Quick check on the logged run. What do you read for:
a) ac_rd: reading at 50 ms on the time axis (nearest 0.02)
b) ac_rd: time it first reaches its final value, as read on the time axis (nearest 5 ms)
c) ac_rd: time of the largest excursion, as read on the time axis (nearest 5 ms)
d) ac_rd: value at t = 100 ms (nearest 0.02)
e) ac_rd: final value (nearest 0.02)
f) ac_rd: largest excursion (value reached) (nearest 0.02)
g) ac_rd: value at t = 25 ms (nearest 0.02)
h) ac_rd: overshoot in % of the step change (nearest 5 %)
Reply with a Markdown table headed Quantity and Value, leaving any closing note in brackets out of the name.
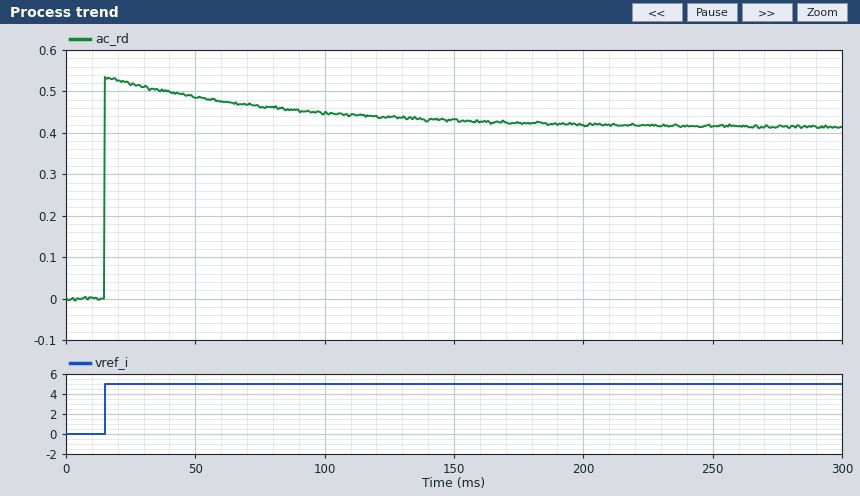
| Quantity | Value |
|---|---|
| ac_rd: reading at 50 ms on the time axis | 0.48 |
| ac_rd: time it first reaches its final value, as read on the time axis | 15 ms |
| ac_rd: time of the largest excursion, as read on the time axis | 15 ms |
| ac_rd: value at t = 100 ms | 0.44 |
| ac_rd: final value | 0.42 |
| ac_rd: largest excursion (value reached) | 0.54 |
| ac_rd: value at t = 25 ms | 0.52 |
| ac_rd: overshoot in % of the step change | 30 % |
